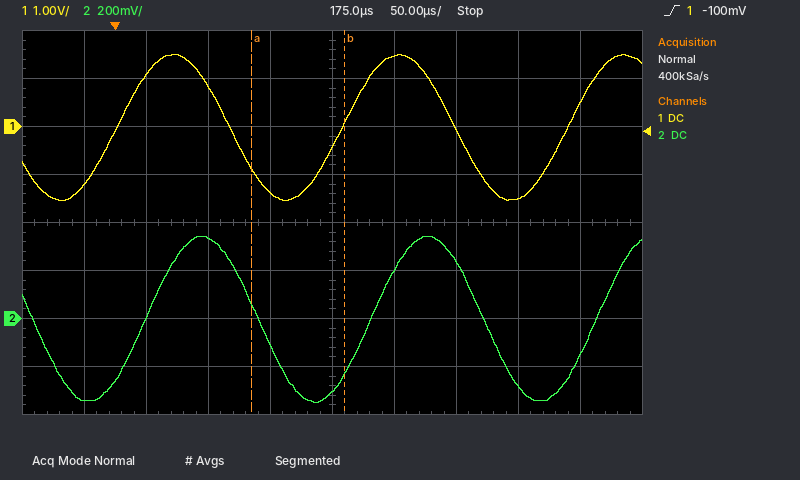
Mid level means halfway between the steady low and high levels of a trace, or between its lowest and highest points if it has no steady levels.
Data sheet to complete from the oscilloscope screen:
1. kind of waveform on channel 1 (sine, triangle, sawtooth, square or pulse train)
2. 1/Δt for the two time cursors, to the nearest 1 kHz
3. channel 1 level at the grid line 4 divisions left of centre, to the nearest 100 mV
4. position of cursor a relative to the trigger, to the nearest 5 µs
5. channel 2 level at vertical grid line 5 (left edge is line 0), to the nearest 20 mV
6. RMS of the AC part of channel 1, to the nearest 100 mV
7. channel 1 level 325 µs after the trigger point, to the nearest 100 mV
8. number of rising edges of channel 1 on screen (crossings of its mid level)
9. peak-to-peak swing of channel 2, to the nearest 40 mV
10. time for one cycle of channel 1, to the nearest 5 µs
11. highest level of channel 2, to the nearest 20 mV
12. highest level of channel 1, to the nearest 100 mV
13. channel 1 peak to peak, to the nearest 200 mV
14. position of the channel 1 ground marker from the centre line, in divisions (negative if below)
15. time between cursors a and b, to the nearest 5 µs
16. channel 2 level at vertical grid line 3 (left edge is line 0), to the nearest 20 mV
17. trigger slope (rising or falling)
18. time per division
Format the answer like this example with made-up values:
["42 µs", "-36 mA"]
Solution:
["sine", "13 kHz", "-1.2 V", "+110 µs", "-300 mV", "1.1 V", "-1.5 V", "3", "680 mV", "180 µs", "340 mV", "1.5 V", "3.0 V", "+2.0 div", "75 µs", "340 mV", "rising", "50 µs"]
